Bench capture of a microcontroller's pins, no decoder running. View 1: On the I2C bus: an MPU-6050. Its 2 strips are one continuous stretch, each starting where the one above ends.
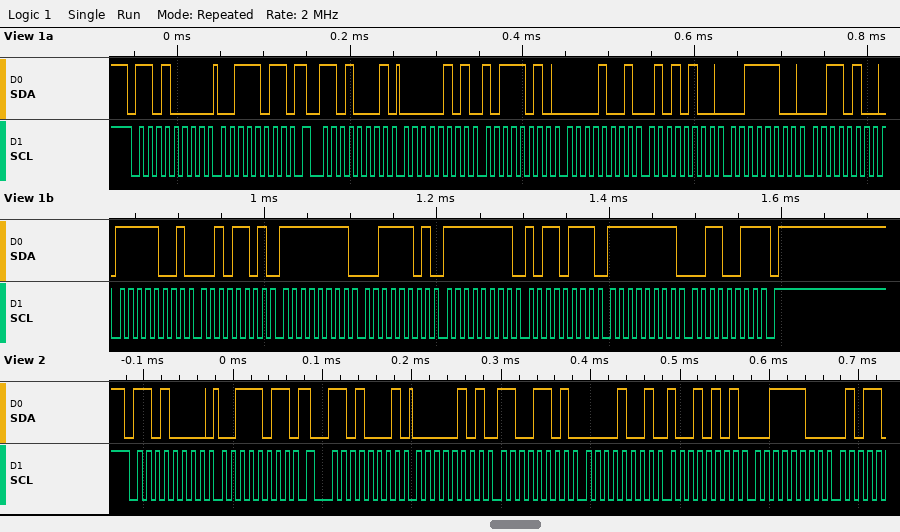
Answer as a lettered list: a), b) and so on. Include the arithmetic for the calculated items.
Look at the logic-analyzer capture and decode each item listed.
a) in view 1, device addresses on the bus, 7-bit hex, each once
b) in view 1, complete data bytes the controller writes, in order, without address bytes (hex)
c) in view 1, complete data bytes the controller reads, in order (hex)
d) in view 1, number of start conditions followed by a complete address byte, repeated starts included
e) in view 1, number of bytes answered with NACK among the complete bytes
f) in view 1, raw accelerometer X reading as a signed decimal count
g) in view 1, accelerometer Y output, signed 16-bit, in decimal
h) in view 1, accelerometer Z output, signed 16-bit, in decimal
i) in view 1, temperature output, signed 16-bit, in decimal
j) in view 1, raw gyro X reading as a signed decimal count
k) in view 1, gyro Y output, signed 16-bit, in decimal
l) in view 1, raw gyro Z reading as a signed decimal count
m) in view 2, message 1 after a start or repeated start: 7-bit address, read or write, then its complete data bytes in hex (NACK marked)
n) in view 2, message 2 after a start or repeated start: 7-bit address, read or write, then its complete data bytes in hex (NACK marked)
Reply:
a) 0x68
b) 3B
c) 05 BA 09 54 3C 34 F9 2D FF 3D FF B7 FF 33
d) 2
e) 1
f) 0x05BA = 1466
g) 0x0954 = 2388
h) 0x3C34 = 15412
i) 0xF92D = -1747
j) 0xFF3D = -195
k) 0xFFB7 = -73
l) 0xFF33 = -205
m) 0x68 write: 3B
n) 0x68 read: 05 CD 09 95 3C
